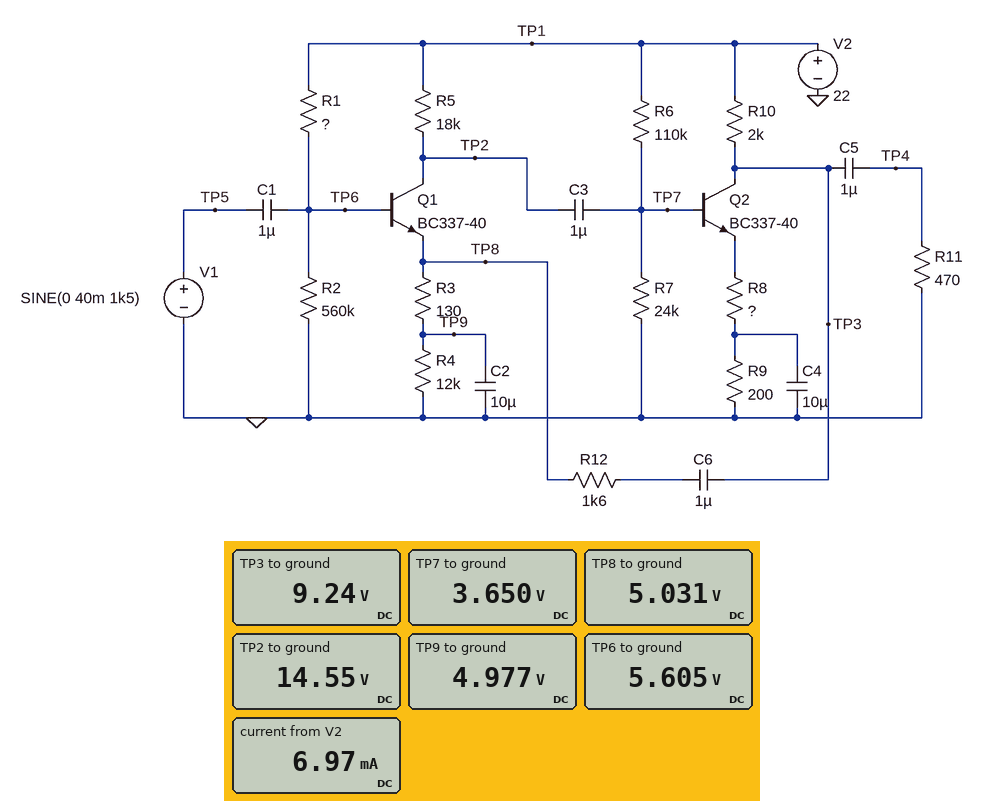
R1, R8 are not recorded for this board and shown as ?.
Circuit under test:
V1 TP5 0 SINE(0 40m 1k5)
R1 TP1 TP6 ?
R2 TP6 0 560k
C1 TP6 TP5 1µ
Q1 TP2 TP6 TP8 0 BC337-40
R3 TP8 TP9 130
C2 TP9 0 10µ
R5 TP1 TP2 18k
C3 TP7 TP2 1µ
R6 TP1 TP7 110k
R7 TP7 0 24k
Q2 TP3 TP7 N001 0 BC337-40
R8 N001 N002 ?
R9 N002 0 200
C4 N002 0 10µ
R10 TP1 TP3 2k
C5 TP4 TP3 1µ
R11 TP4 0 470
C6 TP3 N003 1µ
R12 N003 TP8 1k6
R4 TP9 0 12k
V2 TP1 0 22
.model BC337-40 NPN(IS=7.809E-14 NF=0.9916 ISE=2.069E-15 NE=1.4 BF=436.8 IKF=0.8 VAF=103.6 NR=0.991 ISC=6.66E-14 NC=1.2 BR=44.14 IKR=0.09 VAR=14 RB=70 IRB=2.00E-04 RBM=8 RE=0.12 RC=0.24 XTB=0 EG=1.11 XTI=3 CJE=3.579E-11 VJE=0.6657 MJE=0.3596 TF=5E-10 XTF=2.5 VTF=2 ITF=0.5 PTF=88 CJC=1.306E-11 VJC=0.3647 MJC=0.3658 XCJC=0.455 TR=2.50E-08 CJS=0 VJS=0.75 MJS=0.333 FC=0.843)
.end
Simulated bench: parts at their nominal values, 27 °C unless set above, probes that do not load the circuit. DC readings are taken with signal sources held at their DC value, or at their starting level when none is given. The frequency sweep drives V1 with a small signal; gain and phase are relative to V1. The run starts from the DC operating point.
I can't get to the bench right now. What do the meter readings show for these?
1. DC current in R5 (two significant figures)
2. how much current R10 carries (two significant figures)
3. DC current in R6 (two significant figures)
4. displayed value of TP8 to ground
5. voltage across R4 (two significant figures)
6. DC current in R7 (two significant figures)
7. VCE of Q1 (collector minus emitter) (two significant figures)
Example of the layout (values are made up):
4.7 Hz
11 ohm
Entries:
410 µA
6.4 mA
170 µA
5.031 V
5.0 V
150 µA
9.5 V
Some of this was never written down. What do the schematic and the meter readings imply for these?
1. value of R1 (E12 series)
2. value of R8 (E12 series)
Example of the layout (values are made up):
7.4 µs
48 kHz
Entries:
1.5 MΩ
270 Ω
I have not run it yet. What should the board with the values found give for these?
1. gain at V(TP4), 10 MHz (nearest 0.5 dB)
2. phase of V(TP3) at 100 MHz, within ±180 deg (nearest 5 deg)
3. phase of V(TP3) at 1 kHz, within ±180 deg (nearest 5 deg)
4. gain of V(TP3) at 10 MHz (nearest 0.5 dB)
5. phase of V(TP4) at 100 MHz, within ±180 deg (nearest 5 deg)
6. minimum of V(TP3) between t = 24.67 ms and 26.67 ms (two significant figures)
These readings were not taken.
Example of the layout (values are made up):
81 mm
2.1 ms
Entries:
15.0 dB
95 deg
0 deg
15.0 dB
95 deg
8.8 V
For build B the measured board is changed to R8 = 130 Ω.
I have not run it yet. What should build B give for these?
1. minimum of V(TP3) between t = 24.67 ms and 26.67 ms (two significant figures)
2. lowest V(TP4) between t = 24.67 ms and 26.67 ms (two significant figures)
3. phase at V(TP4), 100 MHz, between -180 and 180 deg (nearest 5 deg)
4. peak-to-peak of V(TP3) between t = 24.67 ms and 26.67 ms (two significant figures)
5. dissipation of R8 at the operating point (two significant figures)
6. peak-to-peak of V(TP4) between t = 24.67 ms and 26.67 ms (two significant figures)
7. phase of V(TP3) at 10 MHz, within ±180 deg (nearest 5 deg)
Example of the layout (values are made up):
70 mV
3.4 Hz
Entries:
4.2 V
-460 mV
100 deg
940 mV
9.8 mW
920 mV
-95 deg
